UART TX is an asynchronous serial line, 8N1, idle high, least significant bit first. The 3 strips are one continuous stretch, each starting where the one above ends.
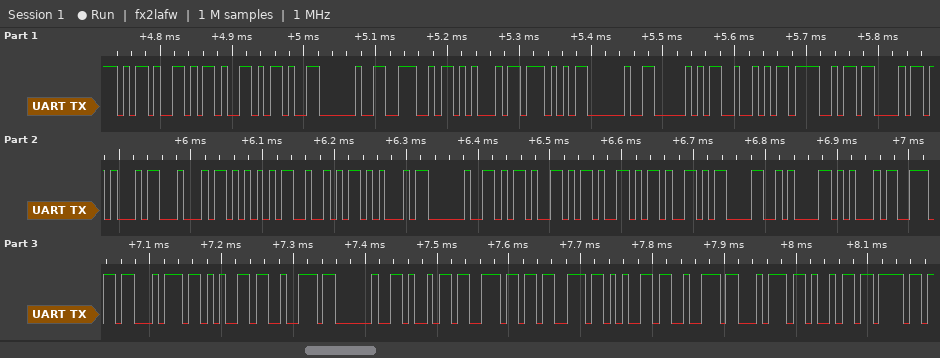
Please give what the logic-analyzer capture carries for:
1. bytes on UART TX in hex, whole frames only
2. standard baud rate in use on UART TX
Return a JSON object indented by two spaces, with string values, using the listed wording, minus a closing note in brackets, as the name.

{
  "bytes on UART TX in hex, whole frames only": "2D 2D 2D 20 4E 45 57 20 50 52 4F 43 45 44 55 52 45 20 2D 2D 2D 0D 0A 45 6E 74 65 72 20 69 6E 73 65 72 74 69 6F",
  "standard baud rate in use on UART TX": "115200 baud"
}
